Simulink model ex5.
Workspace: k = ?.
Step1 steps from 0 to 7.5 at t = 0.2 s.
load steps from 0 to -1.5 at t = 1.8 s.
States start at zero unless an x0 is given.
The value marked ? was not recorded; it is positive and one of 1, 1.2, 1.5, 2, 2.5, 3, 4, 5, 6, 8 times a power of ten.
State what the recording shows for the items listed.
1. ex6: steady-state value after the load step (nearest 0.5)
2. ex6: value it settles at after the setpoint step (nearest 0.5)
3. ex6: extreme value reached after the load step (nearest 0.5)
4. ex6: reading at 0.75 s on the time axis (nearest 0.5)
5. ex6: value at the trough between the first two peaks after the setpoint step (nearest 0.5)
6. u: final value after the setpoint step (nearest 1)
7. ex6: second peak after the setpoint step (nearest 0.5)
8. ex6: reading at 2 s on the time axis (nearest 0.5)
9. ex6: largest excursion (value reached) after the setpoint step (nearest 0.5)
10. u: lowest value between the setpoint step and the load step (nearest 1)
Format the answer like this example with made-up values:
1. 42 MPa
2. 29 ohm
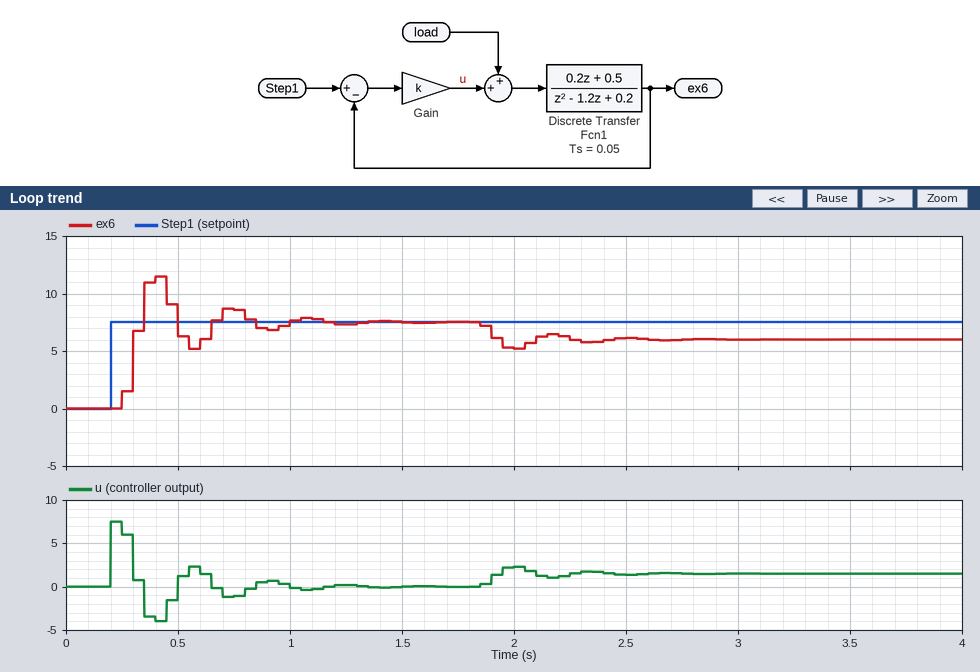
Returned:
1. 6.0
2. 7.5
3. 5.0
4. 8.5
5. 5.0
6. 0
7. 8.5
8. 5.0
9. 11.5
10. -4
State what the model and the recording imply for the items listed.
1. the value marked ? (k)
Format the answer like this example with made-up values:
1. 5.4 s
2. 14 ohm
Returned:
1. 1
